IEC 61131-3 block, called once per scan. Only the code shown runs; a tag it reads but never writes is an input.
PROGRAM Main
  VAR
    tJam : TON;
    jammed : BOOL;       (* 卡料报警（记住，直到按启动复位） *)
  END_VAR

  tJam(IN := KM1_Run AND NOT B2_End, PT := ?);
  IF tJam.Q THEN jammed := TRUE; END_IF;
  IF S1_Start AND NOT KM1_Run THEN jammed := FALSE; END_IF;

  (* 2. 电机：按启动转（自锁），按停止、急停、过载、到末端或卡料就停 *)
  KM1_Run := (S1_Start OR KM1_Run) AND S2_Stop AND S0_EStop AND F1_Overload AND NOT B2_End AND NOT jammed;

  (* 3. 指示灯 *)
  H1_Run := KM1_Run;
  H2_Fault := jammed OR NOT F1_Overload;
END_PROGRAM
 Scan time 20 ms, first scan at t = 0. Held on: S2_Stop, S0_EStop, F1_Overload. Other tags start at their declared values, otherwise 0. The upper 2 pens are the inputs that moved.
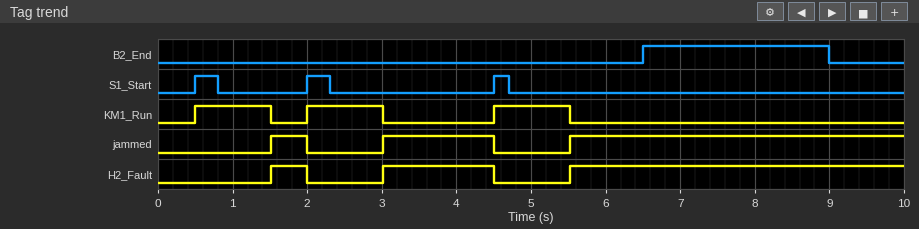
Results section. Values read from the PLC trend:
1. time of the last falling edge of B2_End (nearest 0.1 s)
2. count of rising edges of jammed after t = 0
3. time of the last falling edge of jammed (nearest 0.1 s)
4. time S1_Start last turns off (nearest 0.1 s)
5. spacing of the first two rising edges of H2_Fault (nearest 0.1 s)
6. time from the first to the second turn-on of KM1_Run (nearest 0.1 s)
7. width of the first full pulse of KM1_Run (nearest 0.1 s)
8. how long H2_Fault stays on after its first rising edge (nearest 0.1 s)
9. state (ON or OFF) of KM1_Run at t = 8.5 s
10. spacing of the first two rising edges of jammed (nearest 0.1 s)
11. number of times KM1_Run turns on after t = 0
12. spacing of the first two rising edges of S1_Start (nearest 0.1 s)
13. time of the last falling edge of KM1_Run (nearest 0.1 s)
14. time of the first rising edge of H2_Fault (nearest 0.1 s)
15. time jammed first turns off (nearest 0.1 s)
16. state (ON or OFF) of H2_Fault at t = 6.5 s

9.0 s
3
4.5 s
4.7 s
1.5 s
1.5 s
1.0 s
0.5 s
OFF
1.5 s
3
1.5 s
5.5 s
1.5 s
2.0 s
ON
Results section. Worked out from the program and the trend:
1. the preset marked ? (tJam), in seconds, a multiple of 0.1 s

1.0 s
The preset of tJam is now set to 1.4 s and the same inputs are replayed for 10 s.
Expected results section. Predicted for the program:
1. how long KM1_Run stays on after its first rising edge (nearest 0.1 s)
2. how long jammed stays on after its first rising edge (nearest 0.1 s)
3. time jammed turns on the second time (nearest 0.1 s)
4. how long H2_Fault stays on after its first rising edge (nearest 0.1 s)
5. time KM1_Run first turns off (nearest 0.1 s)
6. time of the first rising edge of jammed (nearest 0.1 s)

1.4 s
0.1 s
3.4 s
0.1 s
1.9 s
1.9 s
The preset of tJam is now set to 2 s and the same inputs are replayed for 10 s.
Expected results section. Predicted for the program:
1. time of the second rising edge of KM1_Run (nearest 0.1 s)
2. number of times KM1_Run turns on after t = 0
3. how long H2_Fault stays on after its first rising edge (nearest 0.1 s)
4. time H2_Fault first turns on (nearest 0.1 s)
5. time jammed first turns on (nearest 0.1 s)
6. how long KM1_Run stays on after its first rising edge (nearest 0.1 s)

4.5 s
2
2.0 s
2.5 s
2.5 s
2.0 s
